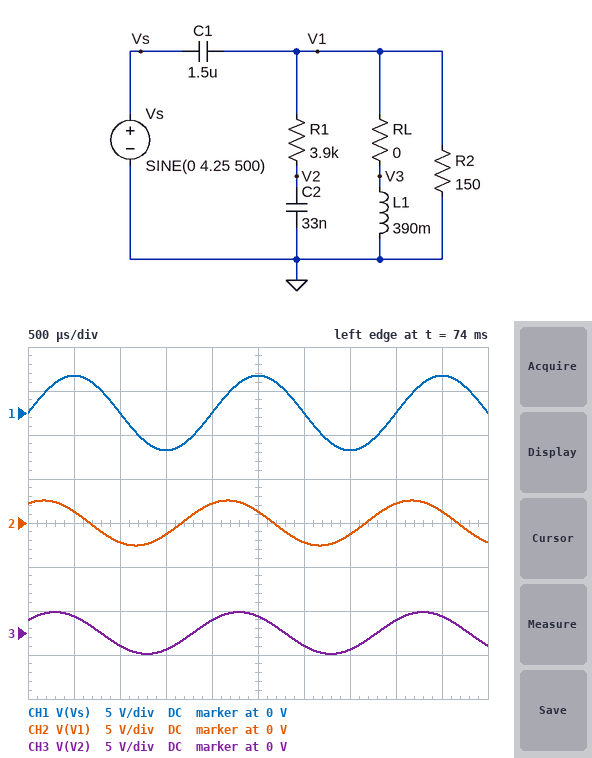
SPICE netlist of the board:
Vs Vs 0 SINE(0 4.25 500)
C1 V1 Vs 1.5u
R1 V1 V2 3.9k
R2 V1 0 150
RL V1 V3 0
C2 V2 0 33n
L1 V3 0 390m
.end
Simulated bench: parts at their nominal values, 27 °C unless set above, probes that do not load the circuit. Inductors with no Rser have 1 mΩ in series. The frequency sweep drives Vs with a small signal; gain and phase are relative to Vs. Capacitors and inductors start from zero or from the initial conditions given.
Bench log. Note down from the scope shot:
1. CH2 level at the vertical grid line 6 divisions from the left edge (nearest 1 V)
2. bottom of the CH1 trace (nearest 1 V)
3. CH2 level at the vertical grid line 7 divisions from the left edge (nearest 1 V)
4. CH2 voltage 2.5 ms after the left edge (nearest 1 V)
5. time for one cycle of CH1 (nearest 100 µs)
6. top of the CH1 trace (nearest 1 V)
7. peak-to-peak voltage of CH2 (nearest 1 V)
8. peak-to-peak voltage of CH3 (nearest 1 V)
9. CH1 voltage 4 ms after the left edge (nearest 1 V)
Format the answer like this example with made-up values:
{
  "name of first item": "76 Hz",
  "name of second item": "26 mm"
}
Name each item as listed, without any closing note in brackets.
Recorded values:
{
  "CH2 level at the vertical grid line 6 divisions from the left edge": "-2 V",
  "bottom of the CH1 trace": "-4 V",
  "CH2 level at the vertical grid line 7 divisions from the left edge": "-1 V",
  "CH2 voltage 2.5 ms after the left edge": "1 V",
  "time for one cycle of CH1": "2.0 ms",
  "top of the CH1 trace": "4 V",
  "peak-to-peak voltage of CH2": "5 V",
  "peak-to-peak voltage of CH3": "5 V",
  "CH1 voltage 4 ms after the left edge": "0 V"
}
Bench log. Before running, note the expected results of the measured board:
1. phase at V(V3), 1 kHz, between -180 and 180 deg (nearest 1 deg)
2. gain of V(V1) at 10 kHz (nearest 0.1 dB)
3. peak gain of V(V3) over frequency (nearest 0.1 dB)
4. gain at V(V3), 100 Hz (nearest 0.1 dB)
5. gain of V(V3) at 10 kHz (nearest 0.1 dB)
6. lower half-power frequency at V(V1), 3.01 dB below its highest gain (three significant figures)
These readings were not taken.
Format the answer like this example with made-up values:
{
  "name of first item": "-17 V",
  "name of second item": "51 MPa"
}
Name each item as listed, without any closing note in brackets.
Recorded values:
{
  "phase at V(V3), 1 kHz, between -180 and 180 deg": "37 deg",
  "gain of V(V1) at 10 kHz": "0 dB",
  "peak gain of V(V3) over frequency": "0 dB",
  "gain at V(V3), 100 Hz": "-17.9 dB",
  "gain of V(V3) at 10 kHz": "0 dB",
  "lower half-power frequency at V(V1), 3.01 dB below its highest gain": "662 Hz"
}
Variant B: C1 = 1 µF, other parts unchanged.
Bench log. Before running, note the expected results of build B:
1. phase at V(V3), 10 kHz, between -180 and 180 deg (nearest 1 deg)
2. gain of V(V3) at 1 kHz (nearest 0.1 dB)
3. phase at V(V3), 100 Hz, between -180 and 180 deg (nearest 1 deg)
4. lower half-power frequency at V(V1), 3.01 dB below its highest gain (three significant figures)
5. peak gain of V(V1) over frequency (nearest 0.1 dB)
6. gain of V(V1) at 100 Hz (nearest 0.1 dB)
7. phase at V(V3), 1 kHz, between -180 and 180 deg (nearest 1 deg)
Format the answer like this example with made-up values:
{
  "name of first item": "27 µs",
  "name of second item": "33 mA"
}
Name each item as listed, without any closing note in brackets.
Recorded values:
{
  "phase at V(V3), 10 kHz, between -180 and 180 deg": "6 deg",
  "gain of V(V3) at 1 kHz": "-3.2 dB",
  "phase at V(V3), 100 Hz, between -180 and 180 deg": "117 deg",
  "lower half-power frequency at V(V1), 3.01 dB below its highest gain": "1.05 kHz",
  "peak gain of V(V1) over frequency": "0 dB",
  "gain of V(V1) at 100 Hz": "-21.6 dB",
  "phase at V(V3), 1 kHz, between -180 and 180 deg": "49 deg"
}
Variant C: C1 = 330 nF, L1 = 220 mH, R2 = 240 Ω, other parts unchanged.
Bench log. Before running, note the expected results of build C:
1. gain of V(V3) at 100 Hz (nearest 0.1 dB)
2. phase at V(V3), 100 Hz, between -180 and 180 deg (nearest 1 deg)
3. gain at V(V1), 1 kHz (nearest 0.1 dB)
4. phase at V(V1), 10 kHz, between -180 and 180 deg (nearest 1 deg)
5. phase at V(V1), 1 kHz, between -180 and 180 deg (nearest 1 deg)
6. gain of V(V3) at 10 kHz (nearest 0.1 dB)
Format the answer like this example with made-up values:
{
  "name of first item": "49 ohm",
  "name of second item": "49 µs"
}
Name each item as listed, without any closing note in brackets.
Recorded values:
{
  "gain of V(V3) at 100 Hz": "-31.9 dB",
  "phase at V(V3), 100 Hz, between -180 and 180 deg": "149 deg",
  "gain at V(V1), 1 kHz": "-6.8 dB",
  "phase at V(V1), 10 kHz, between -180 and 180 deg": "12 deg",
  "phase at V(V1), 1 kHz, between -180 and 180 deg": "71 deg",
  "gain of V(V3) at 10 kHz": "-0.2 dB"
}
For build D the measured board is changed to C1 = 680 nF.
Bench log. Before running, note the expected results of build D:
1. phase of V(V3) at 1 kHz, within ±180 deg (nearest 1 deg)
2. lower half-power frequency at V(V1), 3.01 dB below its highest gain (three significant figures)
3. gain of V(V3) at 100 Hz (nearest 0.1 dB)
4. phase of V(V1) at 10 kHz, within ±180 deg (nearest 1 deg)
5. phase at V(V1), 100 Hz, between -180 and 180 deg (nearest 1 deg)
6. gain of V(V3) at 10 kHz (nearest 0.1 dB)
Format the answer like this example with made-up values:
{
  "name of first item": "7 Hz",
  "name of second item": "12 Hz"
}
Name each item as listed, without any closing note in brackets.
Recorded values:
{
  "phase of V(V3) at 1 kHz, within ±180 deg": "60 deg",
  "lower half-power frequency at V(V1), 3.01 dB below its highest gain": "1.57 kHz",
  "gain of V(V3) at 100 Hz": "-25.0 dB",
  "phase of V(V1) at 10 kHz, within ±180 deg": "9 deg",
  "phase at V(V1), 100 Hz, between -180 and 180 deg": "118 deg",
  "gain of V(V3) at 10 kHz": "-0.1 dB"
}
